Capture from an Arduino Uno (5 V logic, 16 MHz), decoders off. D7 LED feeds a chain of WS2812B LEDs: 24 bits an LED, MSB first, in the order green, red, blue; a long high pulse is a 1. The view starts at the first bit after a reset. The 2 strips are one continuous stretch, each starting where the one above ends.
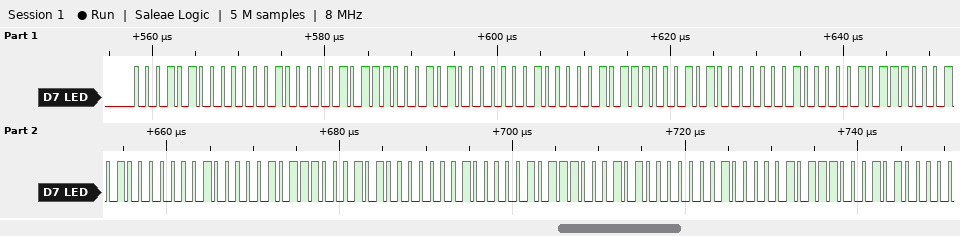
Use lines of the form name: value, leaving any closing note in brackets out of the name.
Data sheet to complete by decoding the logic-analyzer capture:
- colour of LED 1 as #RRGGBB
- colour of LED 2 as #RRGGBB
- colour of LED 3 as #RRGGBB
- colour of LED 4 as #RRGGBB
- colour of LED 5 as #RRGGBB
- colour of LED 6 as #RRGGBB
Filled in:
colour of LED 1 as #RRGGBB: #041417
colour of LED 2 as #RRGGBB: #041417
colour of LED 3 as #RRGGBB: #041417
colour of LED 4 as #RRGGBB: #041417
colour of LED 5 as #RRGGBB: #041417
colour of LED 6 as #RRGGBB: #041417
